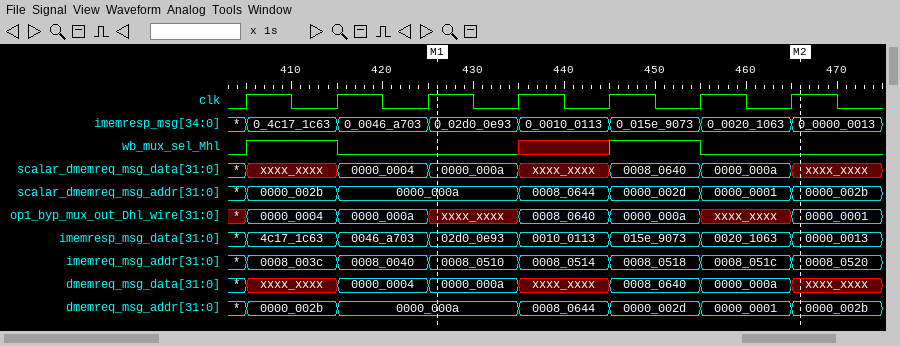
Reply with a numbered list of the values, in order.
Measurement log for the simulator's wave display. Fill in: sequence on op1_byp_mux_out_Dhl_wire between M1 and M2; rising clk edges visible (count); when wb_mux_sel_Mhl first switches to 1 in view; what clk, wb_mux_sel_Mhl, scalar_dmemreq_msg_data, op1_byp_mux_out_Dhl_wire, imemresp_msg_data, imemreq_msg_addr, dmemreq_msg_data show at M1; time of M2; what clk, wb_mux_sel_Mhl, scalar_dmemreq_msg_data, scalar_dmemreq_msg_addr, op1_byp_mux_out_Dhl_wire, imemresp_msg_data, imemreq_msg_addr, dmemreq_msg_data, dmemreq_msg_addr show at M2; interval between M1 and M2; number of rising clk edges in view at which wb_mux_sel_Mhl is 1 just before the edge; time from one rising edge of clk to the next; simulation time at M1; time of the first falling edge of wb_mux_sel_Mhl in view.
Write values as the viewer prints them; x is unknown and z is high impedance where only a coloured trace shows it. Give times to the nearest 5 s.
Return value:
1. xxxx_xxxx, 0008_0640, 0000_000a, xxxx_xxxx, 0000_0001
2. 7
3. 405 s
4. clk=1, wb_mux_sel_Mhl=0, scalar_dmemreq_msg_data=0000_000a, op1_byp_mux_out_Dhl_wire=xxxx_xxxx, imemresp_msg_data=02d0_0e93, imemreq_msg_addr=0008_0510, dmemreq_msg_data=0000_000a
5. 465 s
6. clk=1, wb_mux_sel_Mhl=0, scalar_dmemreq_msg_data=xxxx_xxxx, scalar_dmemreq_msg_addr=0000_002b, op1_byp_mux_out_Dhl_wire=0000_0001, imemresp_msg_data=0000_0013, imemreq_msg_addr=0008_0520, dmemreq_msg_data=xxxx_xxxx, dmemreq_msg_addr=0000_002b
7. 40 s
8. 2
9. 10 s
10. 425 s
11. 415 s
